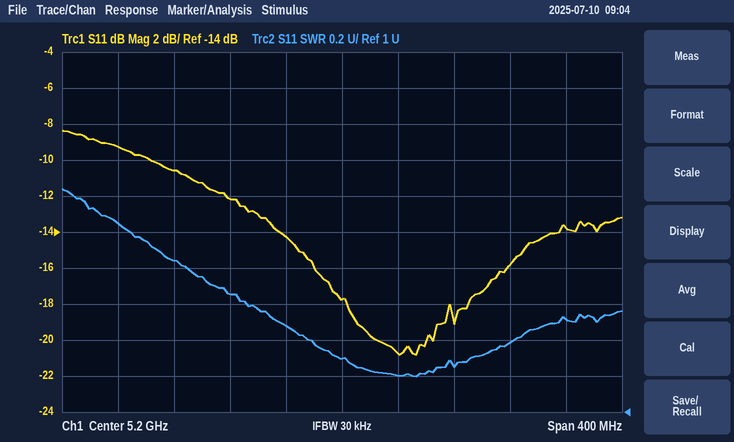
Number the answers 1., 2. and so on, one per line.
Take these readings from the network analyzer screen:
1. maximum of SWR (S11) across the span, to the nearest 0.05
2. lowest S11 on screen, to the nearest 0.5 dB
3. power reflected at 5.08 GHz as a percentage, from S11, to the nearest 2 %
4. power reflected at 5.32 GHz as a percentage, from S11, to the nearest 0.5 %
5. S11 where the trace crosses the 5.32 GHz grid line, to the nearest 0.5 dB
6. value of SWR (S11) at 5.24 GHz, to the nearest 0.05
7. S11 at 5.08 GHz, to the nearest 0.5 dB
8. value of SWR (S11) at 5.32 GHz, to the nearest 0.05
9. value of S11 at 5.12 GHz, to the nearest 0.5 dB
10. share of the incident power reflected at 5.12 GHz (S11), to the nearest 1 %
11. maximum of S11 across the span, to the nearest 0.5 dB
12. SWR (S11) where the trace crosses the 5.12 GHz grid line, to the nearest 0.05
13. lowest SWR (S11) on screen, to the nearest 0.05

1. 2.25
2. -21.0 dB
3. 8 %
4. 2.5 %
5. -16.0 dB
6. 1.20
7. -10.5 dB
8. 1.40
9. -12.0 dB
10. 6 %
11. -8.5 dB
12. 1.65
13. 1.20
